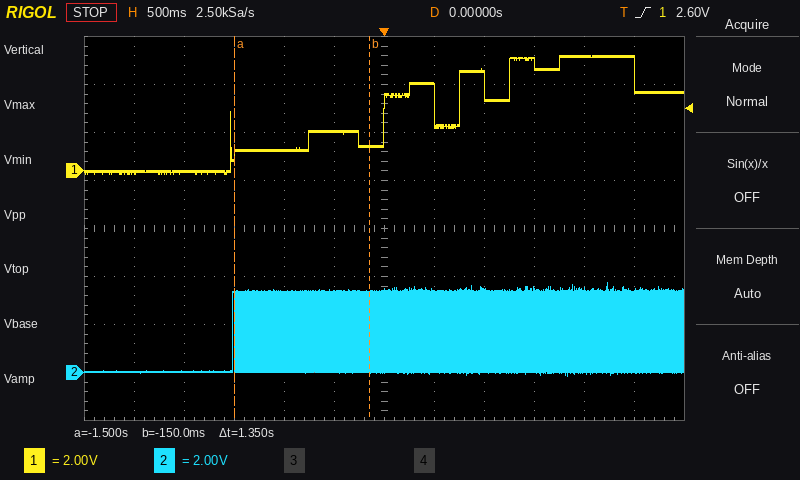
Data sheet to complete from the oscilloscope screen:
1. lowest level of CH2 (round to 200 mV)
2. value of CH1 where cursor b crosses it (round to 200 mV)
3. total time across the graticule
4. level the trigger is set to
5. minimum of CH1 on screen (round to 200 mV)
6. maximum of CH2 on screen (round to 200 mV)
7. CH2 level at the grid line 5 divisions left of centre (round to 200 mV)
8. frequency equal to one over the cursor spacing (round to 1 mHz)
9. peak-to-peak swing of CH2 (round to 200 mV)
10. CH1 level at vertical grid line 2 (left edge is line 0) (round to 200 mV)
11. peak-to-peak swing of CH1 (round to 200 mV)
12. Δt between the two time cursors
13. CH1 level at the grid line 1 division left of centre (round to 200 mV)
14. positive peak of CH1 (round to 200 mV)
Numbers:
-200 mV
1.0 V
6 s
2.60 V
-200 mV
3.8 V
0.0 V
741 mHz
4.0 V
0.0 V
5.0 V
1.35 s
1.6 V
4.8 V
